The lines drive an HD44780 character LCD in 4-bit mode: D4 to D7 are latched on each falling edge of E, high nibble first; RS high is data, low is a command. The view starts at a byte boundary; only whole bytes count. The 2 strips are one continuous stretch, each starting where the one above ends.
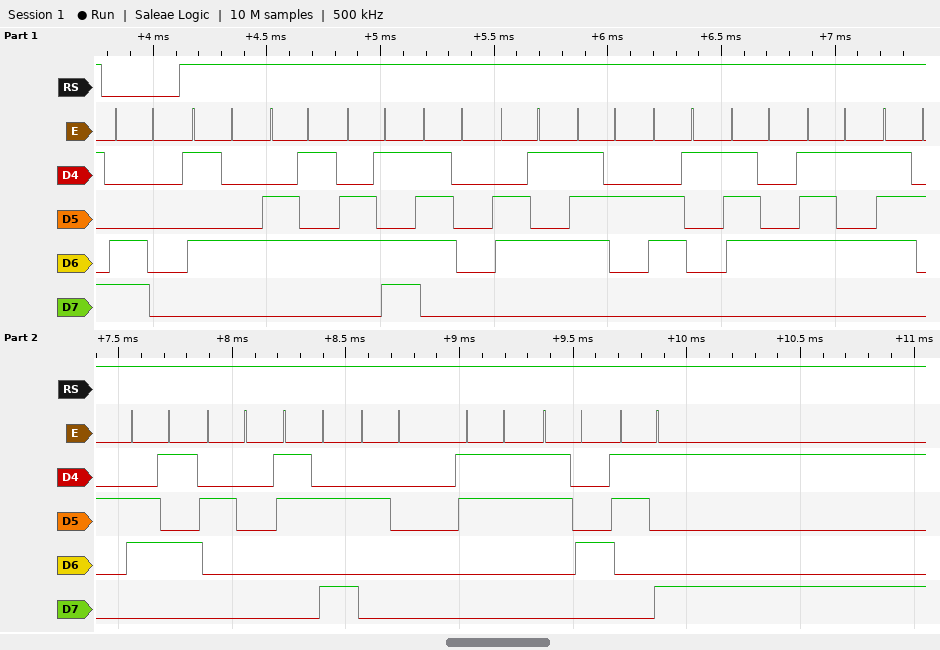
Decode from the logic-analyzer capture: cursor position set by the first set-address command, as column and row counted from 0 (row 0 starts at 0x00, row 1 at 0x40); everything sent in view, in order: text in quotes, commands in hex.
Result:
column 0, row 1
0xC0 "Temperature : 349"
